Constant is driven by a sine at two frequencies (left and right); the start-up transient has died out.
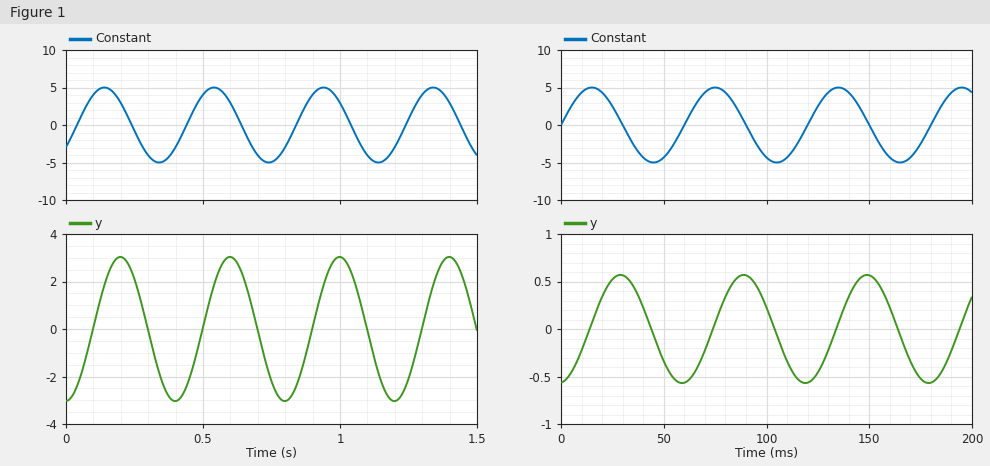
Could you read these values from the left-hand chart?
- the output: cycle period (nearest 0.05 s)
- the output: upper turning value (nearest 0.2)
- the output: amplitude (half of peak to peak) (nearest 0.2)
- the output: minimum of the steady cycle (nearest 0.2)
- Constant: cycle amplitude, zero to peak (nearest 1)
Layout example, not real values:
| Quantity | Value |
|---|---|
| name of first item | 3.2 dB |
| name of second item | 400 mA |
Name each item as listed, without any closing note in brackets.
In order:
| Quantity | Value |
|---|---|
| the output: cycle period | 0.40 s |
| the output: upper turning value | 3.0 |
| the output: amplitude (half of peak to peak) | 3.0 |
| the output: minimum of the steady cycle | -3.0 |
| Constant: cycle amplitude, zero to peak | 5 |
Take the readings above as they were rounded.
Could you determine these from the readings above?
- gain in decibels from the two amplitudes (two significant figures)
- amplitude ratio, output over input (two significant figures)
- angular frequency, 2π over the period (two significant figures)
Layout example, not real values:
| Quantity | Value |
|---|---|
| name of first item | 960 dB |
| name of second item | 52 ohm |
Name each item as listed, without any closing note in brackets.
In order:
| Quantity | Value |
|---|---|
| gain in decibels from the two amplitudes | -4.4 dB |
| amplitude ratio, output over input | 0.60 |
| angular frequency, 2π over the period | 16 rad/s |
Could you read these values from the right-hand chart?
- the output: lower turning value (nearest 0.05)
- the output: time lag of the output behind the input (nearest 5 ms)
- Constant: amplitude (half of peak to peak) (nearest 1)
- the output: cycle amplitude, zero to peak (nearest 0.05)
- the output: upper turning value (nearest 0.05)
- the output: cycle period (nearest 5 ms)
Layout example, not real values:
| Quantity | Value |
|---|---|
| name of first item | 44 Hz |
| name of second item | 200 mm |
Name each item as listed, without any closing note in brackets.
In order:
| Quantity | Value |
|---|---|
| the output: lower turning value | -0.55 |
| the output: time lag of the output behind the input | 15 ms |
| Constant: amplitude (half of peak to peak) | 5 |
| the output: cycle amplitude, zero to peak | 0.55 |
| the output: upper turning value | 0.55 |
| the output: cycle period | 60 ms |
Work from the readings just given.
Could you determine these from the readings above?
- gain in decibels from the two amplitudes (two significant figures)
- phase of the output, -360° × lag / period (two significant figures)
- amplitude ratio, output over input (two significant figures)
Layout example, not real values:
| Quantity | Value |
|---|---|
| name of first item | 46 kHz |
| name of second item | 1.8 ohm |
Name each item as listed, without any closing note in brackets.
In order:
| Quantity | Value |
|---|---|
| gain in decibels from the two amplitudes | -19 dB |
| phase of the output, -360° × lag / period | -90° |
| amplitude ratio, output over input | 0.11 |
